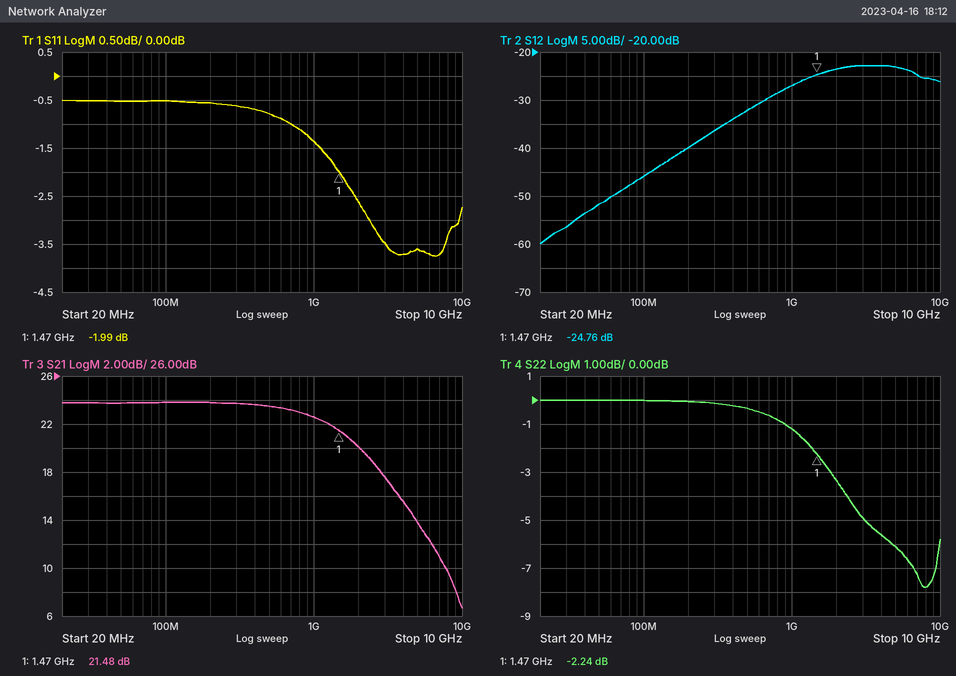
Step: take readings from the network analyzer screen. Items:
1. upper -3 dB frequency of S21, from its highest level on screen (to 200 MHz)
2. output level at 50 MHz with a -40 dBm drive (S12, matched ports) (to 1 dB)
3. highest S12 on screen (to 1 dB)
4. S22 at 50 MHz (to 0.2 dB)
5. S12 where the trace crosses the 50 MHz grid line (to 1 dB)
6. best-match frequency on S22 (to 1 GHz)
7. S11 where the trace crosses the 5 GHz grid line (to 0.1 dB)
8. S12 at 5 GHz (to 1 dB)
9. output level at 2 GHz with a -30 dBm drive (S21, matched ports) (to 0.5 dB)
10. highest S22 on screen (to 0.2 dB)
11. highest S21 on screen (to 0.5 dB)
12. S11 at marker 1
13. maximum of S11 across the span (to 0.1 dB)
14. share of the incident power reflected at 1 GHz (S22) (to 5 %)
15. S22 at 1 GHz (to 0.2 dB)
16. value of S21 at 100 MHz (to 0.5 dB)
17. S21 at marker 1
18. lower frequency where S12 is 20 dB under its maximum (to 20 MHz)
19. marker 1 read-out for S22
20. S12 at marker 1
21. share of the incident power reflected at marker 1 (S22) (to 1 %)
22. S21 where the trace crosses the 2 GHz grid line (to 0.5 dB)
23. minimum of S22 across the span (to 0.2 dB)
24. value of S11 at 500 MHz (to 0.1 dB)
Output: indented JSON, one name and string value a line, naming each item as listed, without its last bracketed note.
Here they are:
{
  "upper -3 dB frequency of S21, from its highest level on screen": "1.8 GHz",
  "output level at 50 MHz with a -40 dBm drive (S12, matched ports)": "-92 dBm",
  "highest S12 on screen": "-23 dB",
  "S22 at 50 MHz": "0.0 dB",
  "S12 where the trace crosses the 50 MHz grid line": "-52 dB",
  "best-match frequency on S22": "8 GHz",
  "S11 where the trace crosses the 5 GHz grid line": "-3.6 dB",
  "S12 at 5 GHz": "-23 dB",
  "output level at 2 GHz with a -30 dBm drive (S21, matched ports)": "-10.0 dBm",
  "highest S22 on screen": "0.0 dB",
  "highest S21 on screen": "24.0 dB",
  "S11 at marker 1": "-1.99 dB",
  "maximum of S11 across the span": "-0.5 dB",
  "share of the incident power reflected at 1 GHz (S22)": "75 %",
  "S22 at 1 GHz": "-1.2 dB",
  "value of S21 at 100 MHz": "24.0 dB",
  "S21 at marker 1": "21.48 dB",
  "lower frequency where S12 is 20 dB under its maximum": "140 MHz",
  "marker 1 read-out for S22": "-2.24 dB",
  "S12 at marker 1": "-24.76 dB",
  "share of the incident power reflected at marker 1 (S22)": "60 %",
  "S21 where the trace crosses the 2 GHz grid line": "20.0 dB",
  "minimum of S22 across the span": "-7.8 dB",
  "value of S11 at 500 MHz": "-0.8 dB"
}
